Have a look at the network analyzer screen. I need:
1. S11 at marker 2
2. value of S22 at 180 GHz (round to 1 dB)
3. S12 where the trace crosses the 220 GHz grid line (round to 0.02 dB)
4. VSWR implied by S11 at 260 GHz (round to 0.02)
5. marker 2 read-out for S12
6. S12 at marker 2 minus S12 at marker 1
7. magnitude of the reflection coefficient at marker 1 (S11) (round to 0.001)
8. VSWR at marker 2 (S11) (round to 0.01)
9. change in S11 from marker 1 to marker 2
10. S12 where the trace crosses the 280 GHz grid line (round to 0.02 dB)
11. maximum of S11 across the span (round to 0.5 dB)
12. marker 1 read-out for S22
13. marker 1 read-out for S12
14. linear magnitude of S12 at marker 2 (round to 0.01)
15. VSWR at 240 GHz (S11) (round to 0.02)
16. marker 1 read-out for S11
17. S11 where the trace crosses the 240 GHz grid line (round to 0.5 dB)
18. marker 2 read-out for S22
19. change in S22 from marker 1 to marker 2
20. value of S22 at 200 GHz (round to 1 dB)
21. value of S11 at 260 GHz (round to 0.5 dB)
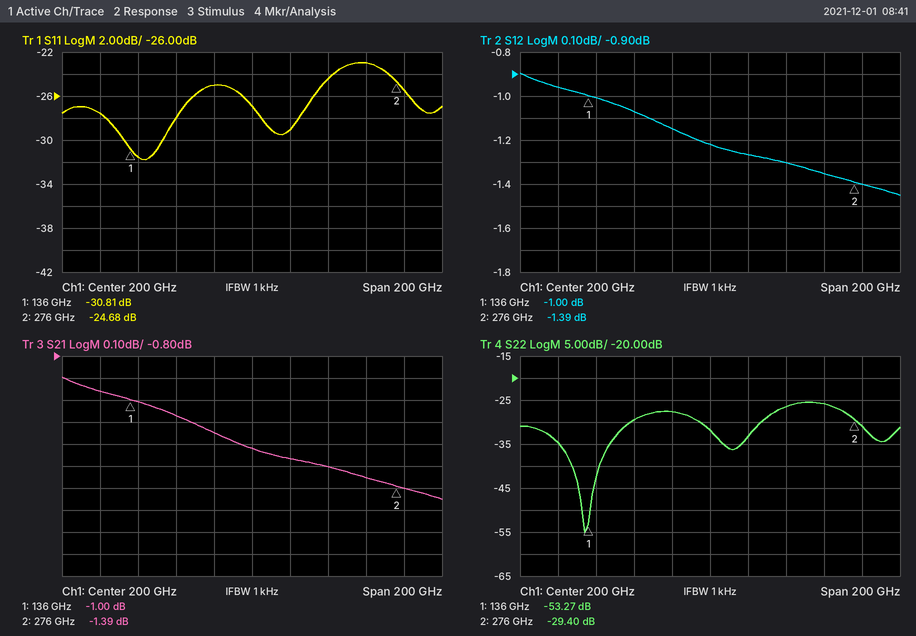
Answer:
-24.68 dB
-28 dB
-1.26 dB
1.16
-1.39 dB
-0.39 dB
0.029
1.12
6.13 dB
-1.40 dB
-23.0 dB
-53.27 dB
-1.00 dB
0.85
1.12
-30.81 dB
-24.5 dB
-29.40 dB
23.87 dB
-32 dB
-23.0 dB
